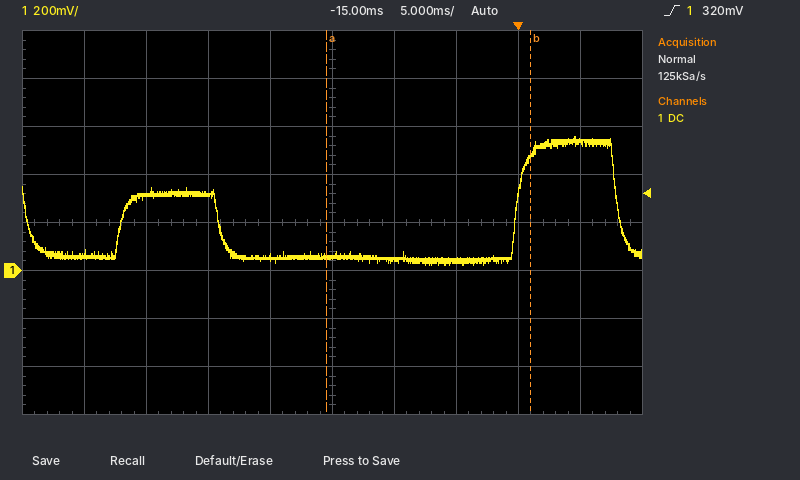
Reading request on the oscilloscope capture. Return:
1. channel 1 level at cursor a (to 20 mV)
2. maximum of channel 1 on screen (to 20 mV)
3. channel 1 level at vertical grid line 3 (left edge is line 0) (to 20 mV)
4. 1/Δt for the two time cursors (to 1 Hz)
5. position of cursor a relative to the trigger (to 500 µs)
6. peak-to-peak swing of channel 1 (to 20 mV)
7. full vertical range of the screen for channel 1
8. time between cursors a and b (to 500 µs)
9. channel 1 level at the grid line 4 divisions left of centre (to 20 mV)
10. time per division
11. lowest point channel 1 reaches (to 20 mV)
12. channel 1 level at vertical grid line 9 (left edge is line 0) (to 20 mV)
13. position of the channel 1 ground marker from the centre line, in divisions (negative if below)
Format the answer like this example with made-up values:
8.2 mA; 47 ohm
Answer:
60 mV; 560 mV; 320 mV; 61 Hz; -15.5 ms; 540 mV; 1.6 V; 16.5 ms; 60 mV; 5 ms; 20 mV; 540 mV; -1.0 div
